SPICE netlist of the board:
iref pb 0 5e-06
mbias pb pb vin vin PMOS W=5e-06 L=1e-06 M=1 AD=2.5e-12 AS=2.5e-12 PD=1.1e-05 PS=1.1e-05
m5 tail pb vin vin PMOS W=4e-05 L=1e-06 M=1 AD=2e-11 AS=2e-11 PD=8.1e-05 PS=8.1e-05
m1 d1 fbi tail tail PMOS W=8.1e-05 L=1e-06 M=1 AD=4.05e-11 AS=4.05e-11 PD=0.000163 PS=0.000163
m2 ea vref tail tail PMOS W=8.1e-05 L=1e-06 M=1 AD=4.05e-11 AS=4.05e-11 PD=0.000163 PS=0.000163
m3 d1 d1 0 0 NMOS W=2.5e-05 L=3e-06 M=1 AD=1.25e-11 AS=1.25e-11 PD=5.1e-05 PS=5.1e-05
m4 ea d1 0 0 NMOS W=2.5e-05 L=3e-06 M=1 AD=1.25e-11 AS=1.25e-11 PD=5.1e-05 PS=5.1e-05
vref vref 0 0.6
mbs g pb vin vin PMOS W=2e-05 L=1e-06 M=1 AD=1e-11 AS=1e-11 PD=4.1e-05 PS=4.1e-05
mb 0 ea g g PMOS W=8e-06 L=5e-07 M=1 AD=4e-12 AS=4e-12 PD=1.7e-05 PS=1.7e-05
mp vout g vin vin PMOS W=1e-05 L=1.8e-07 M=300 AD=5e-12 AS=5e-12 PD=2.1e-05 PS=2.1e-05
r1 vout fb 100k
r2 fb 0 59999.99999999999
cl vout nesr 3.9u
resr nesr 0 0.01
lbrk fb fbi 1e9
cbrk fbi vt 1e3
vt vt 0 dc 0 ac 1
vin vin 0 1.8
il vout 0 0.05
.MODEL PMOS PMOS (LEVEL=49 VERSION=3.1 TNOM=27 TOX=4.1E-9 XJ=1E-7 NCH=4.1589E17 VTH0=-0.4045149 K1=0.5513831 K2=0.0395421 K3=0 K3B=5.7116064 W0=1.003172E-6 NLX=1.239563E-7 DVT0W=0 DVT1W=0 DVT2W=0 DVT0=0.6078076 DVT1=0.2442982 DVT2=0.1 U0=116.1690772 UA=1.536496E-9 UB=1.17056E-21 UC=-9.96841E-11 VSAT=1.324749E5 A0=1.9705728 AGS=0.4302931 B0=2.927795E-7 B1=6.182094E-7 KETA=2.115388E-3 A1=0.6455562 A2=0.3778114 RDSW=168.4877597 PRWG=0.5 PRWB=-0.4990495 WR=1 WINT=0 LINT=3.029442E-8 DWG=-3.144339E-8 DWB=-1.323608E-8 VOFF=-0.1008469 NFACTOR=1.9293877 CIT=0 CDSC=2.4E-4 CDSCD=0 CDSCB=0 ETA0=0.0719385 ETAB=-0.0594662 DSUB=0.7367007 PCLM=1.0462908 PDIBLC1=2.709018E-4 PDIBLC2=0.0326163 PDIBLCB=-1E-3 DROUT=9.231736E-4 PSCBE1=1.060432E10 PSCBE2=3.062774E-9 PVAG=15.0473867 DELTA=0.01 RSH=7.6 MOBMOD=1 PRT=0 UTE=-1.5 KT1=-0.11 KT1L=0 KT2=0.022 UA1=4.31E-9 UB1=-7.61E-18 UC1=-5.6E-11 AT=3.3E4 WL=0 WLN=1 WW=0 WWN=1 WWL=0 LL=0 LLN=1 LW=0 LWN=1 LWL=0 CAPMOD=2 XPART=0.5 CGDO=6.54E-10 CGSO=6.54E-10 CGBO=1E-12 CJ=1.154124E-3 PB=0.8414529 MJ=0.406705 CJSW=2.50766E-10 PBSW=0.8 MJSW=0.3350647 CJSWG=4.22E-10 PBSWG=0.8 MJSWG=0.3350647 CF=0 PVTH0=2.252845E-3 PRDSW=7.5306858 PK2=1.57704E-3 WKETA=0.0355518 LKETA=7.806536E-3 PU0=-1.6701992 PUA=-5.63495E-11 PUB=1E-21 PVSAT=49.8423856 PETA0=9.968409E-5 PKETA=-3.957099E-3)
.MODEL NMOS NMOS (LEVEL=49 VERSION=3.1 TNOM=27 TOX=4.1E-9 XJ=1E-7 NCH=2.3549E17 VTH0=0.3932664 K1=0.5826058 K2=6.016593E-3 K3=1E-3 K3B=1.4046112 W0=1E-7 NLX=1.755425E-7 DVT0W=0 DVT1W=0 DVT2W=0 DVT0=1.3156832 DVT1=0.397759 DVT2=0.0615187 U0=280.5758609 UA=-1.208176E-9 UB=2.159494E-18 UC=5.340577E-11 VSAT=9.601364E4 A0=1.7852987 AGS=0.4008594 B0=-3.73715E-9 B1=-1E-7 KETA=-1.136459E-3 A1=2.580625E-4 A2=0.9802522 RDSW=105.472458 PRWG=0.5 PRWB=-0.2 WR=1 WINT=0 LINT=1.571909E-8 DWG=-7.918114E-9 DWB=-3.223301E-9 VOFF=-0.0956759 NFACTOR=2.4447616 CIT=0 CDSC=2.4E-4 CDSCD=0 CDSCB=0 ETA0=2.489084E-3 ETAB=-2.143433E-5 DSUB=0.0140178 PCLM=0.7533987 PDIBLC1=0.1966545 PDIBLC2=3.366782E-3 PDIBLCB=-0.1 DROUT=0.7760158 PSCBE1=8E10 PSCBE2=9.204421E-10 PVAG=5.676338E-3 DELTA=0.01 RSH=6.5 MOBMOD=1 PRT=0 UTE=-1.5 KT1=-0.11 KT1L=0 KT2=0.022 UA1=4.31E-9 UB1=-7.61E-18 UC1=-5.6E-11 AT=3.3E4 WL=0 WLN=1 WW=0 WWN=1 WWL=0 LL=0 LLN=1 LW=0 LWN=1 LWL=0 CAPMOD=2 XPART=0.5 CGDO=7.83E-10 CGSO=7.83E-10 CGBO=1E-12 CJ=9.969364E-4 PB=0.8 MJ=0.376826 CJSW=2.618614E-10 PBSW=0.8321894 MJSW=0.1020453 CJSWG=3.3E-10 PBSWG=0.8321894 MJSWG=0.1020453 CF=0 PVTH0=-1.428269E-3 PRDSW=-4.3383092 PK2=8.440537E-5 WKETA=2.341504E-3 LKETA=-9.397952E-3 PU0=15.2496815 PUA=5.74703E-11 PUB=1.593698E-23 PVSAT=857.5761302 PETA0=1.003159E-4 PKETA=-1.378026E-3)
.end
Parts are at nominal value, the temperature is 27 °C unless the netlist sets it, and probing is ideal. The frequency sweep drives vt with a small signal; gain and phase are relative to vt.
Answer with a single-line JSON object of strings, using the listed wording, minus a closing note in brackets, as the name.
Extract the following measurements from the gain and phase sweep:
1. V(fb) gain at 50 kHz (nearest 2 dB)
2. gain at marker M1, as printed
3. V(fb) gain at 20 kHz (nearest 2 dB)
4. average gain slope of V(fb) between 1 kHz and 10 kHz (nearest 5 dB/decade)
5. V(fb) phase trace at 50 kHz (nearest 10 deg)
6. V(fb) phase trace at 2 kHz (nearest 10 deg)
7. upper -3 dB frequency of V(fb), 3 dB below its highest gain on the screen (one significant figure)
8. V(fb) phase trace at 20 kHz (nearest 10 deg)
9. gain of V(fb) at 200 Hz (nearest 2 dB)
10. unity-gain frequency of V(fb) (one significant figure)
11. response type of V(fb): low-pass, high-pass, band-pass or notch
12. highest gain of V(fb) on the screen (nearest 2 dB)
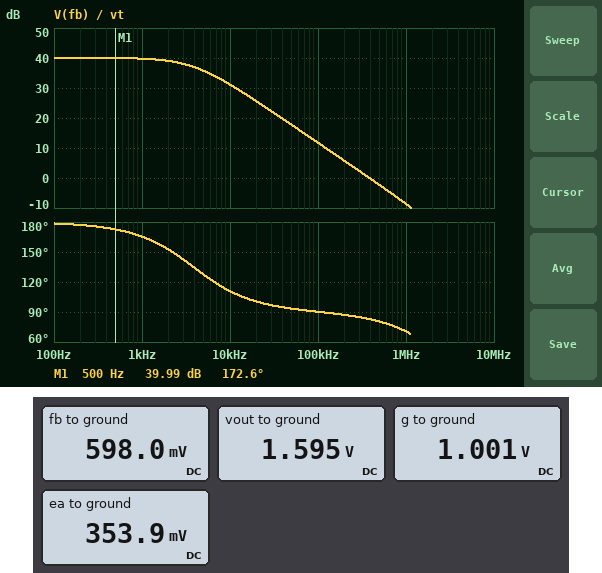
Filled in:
{"V(fb) gain at 50 kHz": "18 dB", "gain at marker M1, as printed": "39.99 dB", "V(fb) gain at 20 kHz": "26 dB", "average gain slope of V(fb) between 1 kHz and 10 kHz": "-10 dB/decade", "V(fb) phase trace at 50 kHz": "90 deg", "V(fb) phase trace at 2 kHz": "150 deg", "upper -3 dB frequency of V(fb), 3 dB below its highest gain on the screen": "4 kHz", "V(fb) phase trace at 20 kHz": "100 deg", "gain of V(fb) at 200 Hz": "40 dB", "unity-gain frequency of V(fb)": "400 kHz", "response type of V(fb): low-pass, high-pass, band-pass or notch": "low-pass", "highest gain of V(fb) on the screen": "40 dB"}
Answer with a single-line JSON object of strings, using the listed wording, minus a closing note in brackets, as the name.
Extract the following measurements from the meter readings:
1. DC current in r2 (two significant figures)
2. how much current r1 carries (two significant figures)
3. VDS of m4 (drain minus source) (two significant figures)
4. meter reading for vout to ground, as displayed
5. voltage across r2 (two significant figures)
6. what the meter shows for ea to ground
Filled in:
{"DC current in r2": "10 µA", "how much current r1 carries": "10 µA", "VDS of m4 (drain minus source)": "350 mV", "meter reading for vout to ground, as displayed": "1.595 V", "voltage across r2": "600 mV", "what the meter shows for ea to ground": "353.9 mV"}
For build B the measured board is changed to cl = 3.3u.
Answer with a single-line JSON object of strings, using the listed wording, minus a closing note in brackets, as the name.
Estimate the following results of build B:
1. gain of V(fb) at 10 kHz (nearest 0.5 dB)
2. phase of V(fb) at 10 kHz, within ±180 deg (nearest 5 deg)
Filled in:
{"gain of V(fb) at 10 kHz": "32.5 dB", "phase of V(fb) at 10 kHz, within ±180 deg": "115 deg"}
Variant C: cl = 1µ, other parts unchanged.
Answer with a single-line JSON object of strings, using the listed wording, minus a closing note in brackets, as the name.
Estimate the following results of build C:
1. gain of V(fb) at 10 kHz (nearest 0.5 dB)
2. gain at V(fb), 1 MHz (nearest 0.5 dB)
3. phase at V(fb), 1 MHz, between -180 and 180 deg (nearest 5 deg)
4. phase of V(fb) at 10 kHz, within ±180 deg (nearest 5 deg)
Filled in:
{"gain of V(fb) at 10 kHz": "38.5 dB", "gain at V(fb), 1 MHz": "3.0 dB", "phase at V(fb), 1 MHz, between -180 and 180 deg": "60 deg", "phase of V(fb) at 10 kHz, within ±180 deg": "145 deg"}
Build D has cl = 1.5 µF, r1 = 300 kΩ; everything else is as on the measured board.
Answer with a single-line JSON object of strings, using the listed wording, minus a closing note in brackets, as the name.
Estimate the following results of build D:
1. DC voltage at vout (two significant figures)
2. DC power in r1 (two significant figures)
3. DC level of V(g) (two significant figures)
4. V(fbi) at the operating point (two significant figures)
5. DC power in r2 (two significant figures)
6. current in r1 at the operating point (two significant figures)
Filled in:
{"DC voltage at vout": "1.7 V", "DC power in r1": "7.0 µW", "DC level of V(g)": "650 mV", "V(fbi) at the operating point": "290 mV", "DC power in r2": "1.4 µW", "current in r1 at the operating point": "4.8 µA"}
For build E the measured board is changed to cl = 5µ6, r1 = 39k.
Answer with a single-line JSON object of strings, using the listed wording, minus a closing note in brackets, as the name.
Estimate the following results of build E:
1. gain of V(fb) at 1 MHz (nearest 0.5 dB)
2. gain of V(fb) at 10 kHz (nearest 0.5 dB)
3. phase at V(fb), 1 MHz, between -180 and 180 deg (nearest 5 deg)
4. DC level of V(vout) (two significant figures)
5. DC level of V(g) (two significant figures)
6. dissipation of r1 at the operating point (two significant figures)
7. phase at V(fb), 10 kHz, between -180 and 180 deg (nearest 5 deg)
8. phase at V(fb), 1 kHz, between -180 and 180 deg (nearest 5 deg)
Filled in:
{"gain of V(fb) at 1 MHz": "-5.0 dB", "gain of V(fb) at 10 kHz": "35.0 dB", "phase at V(fb), 1 MHz, between -180 and 180 deg": "75 deg", "DC level of V(vout)": "990 mV", "DC level of V(g)": "1.0 V", "dissipation of r1 at the operating point": "3.9 µW", "phase at V(fb), 10 kHz, between -180 and 180 deg": "90 deg", "phase at V(fb), 1 kHz, between -180 and 180 deg": "110 deg"}
